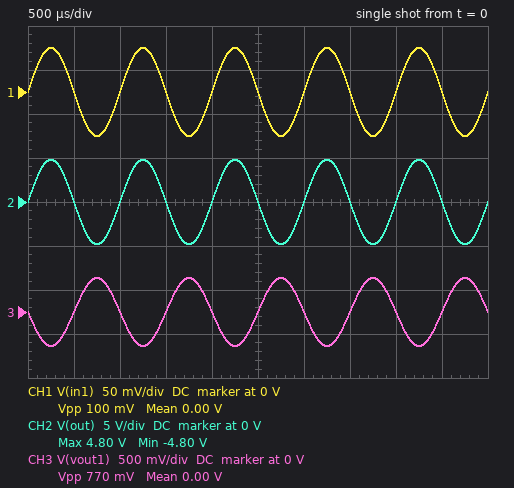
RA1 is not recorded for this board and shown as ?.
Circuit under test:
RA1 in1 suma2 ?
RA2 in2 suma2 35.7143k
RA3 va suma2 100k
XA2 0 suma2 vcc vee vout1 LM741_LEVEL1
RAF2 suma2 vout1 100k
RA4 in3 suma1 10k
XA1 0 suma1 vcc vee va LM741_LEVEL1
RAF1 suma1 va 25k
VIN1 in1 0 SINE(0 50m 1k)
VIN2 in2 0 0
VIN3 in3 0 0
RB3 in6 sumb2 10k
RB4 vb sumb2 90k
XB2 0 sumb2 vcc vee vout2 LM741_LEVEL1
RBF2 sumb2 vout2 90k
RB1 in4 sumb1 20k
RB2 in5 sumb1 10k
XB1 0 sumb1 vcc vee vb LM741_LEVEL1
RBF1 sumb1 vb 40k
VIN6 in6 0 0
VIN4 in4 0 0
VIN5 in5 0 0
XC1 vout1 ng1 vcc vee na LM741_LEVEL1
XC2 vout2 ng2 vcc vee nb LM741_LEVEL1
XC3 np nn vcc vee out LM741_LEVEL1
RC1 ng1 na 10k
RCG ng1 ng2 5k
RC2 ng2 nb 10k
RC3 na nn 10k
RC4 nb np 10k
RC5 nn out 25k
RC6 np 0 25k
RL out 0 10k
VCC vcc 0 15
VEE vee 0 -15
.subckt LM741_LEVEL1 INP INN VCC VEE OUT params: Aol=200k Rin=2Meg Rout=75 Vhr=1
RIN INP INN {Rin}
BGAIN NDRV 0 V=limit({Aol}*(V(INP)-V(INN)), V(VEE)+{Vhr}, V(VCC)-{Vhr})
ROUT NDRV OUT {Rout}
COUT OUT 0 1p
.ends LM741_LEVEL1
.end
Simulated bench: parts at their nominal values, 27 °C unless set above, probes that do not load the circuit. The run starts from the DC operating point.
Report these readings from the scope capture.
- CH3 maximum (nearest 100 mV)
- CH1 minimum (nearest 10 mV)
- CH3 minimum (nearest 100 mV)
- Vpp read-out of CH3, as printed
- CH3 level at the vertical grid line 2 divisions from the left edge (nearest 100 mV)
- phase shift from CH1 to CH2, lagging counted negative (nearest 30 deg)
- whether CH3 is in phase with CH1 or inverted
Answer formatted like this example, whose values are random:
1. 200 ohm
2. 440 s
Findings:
1. 400 mV
2. -50 mV
3. -400 mV
4. 770 mV
5. 0 V
6. 0 deg
7. inverted
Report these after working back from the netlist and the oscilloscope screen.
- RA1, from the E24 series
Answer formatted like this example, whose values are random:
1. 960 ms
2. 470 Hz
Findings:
1. 13 kΩ
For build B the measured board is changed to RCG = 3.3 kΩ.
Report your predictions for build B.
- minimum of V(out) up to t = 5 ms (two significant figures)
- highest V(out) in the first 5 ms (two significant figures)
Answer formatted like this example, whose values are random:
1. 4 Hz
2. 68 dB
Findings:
1. -6.8 V
2. 6.8 V
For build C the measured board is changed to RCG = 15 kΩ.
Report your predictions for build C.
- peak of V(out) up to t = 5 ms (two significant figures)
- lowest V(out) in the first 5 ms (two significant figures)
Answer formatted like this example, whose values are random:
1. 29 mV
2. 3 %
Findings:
1. 2.2 V
2. -2.2 V
